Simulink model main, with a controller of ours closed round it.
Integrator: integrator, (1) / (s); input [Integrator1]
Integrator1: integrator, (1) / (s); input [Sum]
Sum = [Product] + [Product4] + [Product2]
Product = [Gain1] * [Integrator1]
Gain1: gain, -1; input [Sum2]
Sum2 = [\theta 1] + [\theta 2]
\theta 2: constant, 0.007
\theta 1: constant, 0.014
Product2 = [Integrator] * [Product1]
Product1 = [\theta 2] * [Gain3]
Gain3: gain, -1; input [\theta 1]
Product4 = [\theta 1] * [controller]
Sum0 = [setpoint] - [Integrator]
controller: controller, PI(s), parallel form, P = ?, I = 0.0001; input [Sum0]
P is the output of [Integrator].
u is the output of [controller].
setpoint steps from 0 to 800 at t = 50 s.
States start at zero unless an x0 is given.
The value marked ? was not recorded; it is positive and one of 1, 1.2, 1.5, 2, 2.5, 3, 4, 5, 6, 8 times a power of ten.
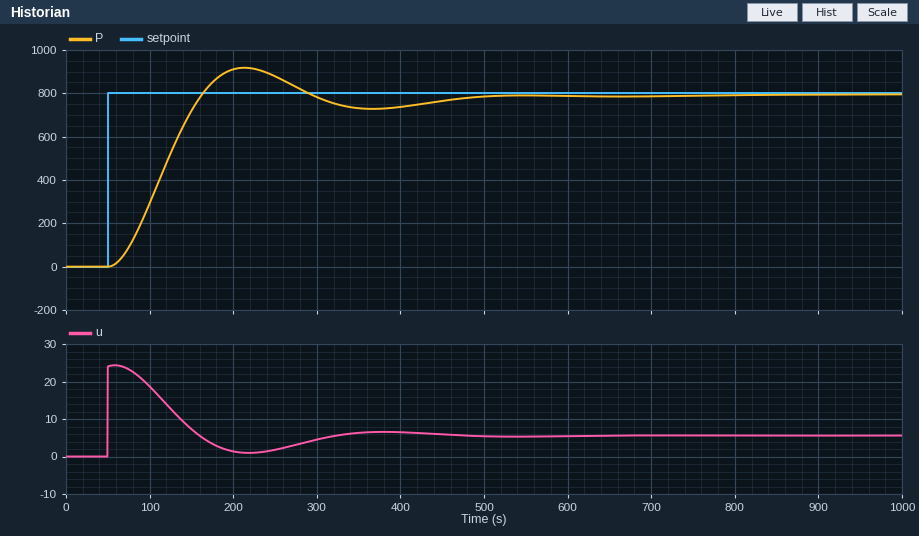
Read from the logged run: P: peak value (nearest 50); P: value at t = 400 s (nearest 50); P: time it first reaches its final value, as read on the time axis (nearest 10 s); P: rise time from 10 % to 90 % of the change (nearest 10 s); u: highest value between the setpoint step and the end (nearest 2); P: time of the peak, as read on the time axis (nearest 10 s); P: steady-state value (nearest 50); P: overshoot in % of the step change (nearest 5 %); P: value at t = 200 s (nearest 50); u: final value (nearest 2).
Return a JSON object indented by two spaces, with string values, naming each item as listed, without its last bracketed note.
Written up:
{
  "P: peak value": "900",
  "P: value at t = 400 s": "750",
  "P: time it first reaches its final value, as read on the time axis": "160 s",
  "P: rise time from 10 % to 90 % of the change": "80 s",
  "u: highest value between the setpoint step and the end": "24",
  "P: time of the peak, as read on the time axis": "210 s",
  "P: steady-state value": "800",
  "P: overshoot in % of the step change": "15 %",
  "P: value at t = 200 s": "900",
  "u: final value": "6"
}
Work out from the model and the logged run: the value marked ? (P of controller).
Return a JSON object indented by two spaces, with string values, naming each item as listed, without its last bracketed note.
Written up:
{
  "the value marked ?": "0.03"
}
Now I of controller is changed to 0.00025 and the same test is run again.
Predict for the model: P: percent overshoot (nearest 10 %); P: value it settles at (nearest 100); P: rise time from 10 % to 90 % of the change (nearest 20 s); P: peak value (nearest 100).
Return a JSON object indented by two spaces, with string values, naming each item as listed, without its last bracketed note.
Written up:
{
  "P: percent overshoot": "40 %",
  "P: value it settles at": "800",
  "P: rise time from 10 % to 90 % of the change": "60 s",
  "P: peak value": "1100"
}
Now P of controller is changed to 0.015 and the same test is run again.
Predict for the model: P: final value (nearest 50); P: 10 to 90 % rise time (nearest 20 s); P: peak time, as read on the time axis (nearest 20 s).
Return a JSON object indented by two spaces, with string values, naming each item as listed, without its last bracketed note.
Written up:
{
  "P: final value": "800",
  "P: 10 to 90 % rise time": "120 s",
  "P: peak time, as read on the time axis": "300 s"
}
